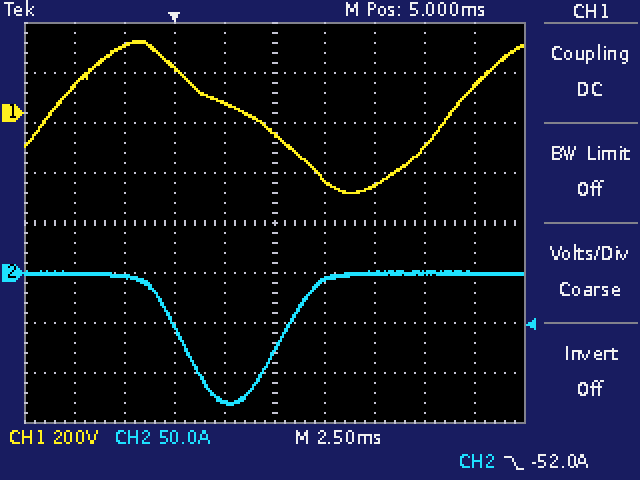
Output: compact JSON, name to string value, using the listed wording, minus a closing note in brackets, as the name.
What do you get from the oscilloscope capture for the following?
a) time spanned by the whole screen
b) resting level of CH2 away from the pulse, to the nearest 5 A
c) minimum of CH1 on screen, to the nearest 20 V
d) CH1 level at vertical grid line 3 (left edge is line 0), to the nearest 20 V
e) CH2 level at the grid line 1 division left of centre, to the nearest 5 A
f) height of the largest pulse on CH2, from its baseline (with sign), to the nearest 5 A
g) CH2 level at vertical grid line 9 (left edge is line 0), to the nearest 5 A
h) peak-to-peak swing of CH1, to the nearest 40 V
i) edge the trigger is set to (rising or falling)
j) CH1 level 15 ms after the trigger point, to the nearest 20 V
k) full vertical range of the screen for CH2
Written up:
{"time spanned by the whole screen": "25 ms", "resting level of CH2 away from the pulse, to the nearest 5 A": "0 A", "minimum of CH1 on screen, to the nearest 20 V": "-320 V", "CH1 level at vertical grid line 3 (left edge is line 0), to the nearest 20 V": "180 V", "CH2 level at the grid line 1 division left of centre, to the nearest 5 A": "-130 A", "height of the largest pulse on CH2, from its baseline (with sign), to the nearest 5 A": "-130 A", "CH2 level at vertical grid line 9 (left edge is line 0), to the nearest 5 A": "0 A", "peak-to-peak swing of CH1, to the nearest 40 V": "600 V", "edge the trigger is set to": "falling", "CH1 level 15 ms after the trigger point, to the nearest 20 V": "100 V", "full vertical range of the screen for CH2": "400 A"}
